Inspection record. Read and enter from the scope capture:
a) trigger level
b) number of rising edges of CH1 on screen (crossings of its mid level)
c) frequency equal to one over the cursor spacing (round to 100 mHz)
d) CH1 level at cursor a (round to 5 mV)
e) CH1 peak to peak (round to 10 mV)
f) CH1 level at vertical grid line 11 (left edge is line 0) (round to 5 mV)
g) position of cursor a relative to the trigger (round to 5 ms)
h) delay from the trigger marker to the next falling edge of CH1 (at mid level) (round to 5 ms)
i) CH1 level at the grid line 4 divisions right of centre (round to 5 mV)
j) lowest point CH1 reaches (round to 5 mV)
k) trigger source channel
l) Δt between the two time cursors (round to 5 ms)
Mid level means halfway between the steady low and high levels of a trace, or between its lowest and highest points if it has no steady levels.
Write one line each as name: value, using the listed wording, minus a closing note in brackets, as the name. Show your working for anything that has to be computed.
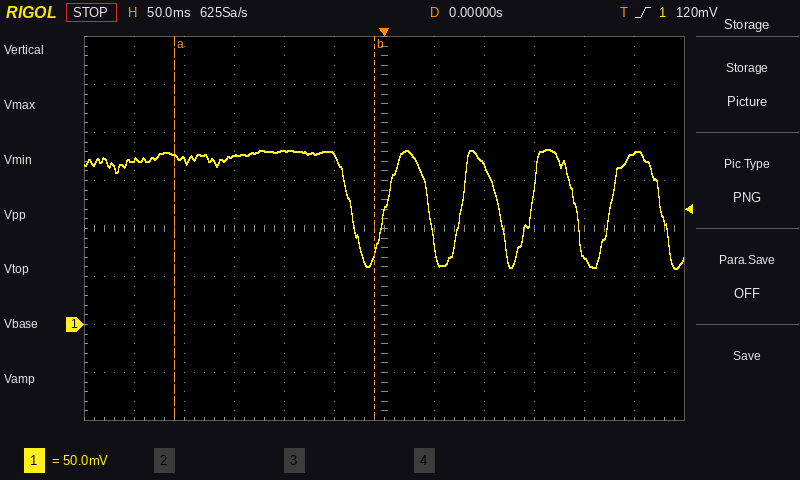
trigger level: 120 mV
number of rising edges of CH1 on screen: 4
frequency equal to one over the cursor spacing: 1 / 200 ms ≈ 5.0 Hz
CH1 level at cursor a: 175 mV
CH1 peak to peak: 120 mV
CH1 level at vertical grid line 11 (left edge is line 0): 180 mV
position of cursor a relative to the trigger: -210 ms
delay from the trigger marker to the next falling edge of CH1 (at mid level): 45 ms
CH1 level at the grid line 4 divisions right of centre: 70 mV
lowest point CH1 reaches: 60 mV
trigger source channel: CH1
Δt between the two time cursors: 200 ms
